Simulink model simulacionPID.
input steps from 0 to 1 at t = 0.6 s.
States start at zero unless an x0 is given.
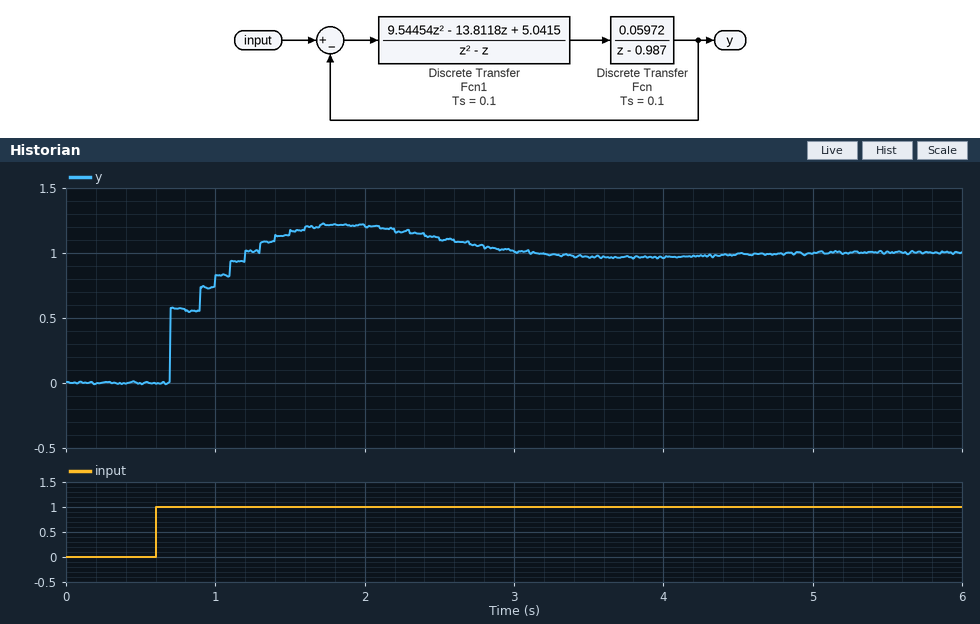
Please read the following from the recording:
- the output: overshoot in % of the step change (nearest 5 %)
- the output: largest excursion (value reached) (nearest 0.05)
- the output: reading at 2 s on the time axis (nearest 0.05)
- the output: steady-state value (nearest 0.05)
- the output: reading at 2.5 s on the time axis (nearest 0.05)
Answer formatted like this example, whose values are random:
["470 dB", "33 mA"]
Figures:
["20 %", "1.20", "1.20", "1.00", "1.10"]
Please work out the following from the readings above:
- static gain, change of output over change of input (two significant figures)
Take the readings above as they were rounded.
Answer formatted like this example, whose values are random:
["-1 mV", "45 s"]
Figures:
["1.0"]
